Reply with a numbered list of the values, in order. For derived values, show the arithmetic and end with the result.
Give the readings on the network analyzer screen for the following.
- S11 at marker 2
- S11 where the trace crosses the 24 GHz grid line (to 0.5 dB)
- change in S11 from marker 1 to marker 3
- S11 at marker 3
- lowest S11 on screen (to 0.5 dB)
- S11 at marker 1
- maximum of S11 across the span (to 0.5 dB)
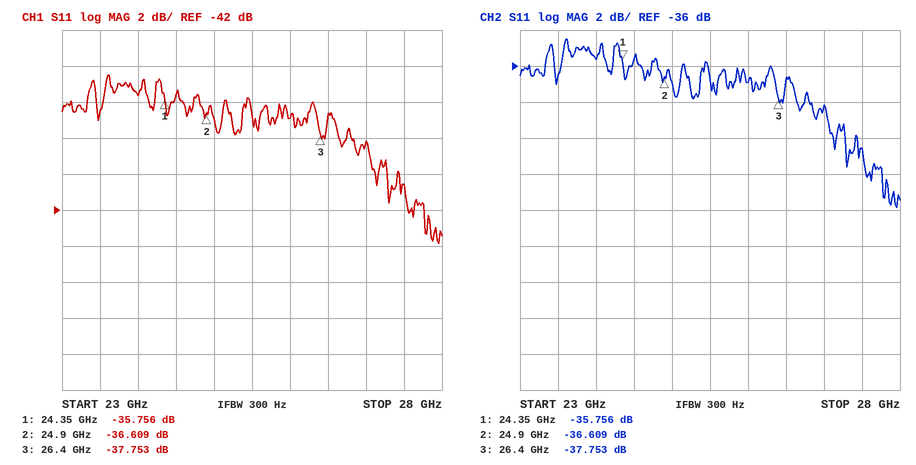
1. -36.609 dB
2. -35.5 dB
3. -37.753 − (-35.756) = -1.997 dB
4. -37.753 dB
5. -44.0 dB
6. -35.756 dB
7. -34.5 dB
